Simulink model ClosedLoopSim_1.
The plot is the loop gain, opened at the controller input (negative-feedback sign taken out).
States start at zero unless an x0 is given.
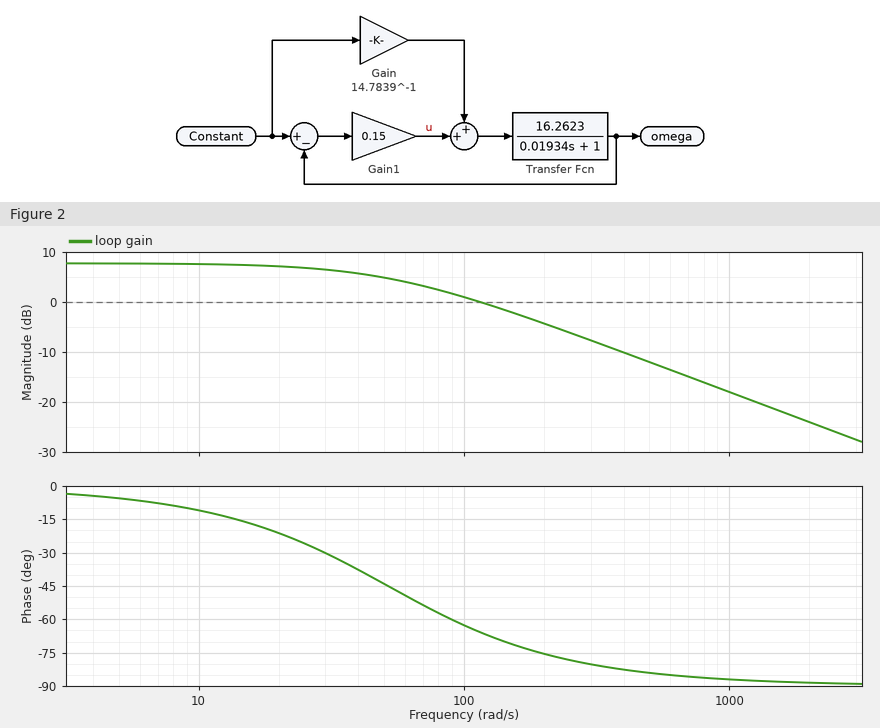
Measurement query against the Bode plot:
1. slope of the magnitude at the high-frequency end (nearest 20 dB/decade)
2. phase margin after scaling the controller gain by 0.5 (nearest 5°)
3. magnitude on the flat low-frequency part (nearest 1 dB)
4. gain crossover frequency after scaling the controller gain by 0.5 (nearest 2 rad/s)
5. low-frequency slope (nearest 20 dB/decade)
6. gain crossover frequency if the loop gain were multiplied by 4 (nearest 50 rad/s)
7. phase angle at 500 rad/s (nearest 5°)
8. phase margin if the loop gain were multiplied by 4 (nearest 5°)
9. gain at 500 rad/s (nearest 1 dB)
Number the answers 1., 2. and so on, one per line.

1. -20 dB/decade
2. 145°
3. 8 dB
4. 36 rad/s
5. 0 dB/decade
6. 500 rad/s
7. -85°
8. 95°
9. -12 dB
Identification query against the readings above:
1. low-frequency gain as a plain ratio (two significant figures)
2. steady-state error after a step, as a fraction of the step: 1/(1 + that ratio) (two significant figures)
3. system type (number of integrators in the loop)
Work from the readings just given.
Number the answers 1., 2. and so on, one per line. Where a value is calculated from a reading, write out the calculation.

1. 10^(8 / 20) = 2.5
2. 1 / (1 + 2.5) = 0.29
3. 0
